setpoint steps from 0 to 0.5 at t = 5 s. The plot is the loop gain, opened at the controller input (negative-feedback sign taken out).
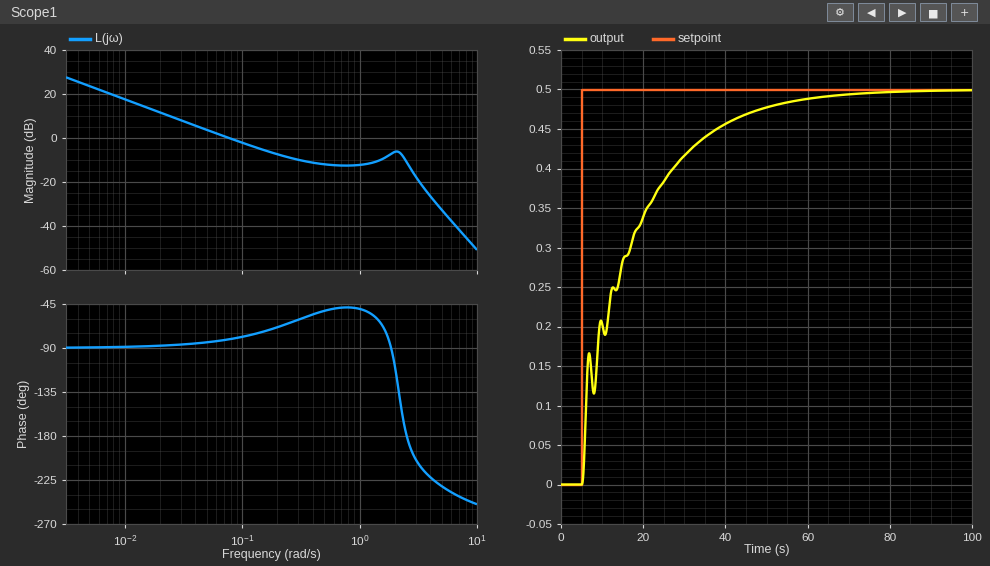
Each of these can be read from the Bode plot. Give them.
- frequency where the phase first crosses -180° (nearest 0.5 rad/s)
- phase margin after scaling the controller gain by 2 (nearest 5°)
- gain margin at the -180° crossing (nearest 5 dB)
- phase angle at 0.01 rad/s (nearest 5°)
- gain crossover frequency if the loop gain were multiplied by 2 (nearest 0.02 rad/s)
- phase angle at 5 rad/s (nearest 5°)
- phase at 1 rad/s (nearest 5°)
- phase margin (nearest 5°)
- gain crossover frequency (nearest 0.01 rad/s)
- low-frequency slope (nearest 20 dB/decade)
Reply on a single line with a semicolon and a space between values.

2.5 rad/s; 110°; 10 dB; -90°; 0.16 rad/s; -230°; -50°; 100°; 0.08 rad/s; -20 dB/decade
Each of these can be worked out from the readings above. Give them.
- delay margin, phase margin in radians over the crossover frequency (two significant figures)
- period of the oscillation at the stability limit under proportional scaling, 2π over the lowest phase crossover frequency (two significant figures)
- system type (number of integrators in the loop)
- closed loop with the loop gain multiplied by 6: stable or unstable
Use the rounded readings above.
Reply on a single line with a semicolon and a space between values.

22 s; 2.5 s; 1; unstable
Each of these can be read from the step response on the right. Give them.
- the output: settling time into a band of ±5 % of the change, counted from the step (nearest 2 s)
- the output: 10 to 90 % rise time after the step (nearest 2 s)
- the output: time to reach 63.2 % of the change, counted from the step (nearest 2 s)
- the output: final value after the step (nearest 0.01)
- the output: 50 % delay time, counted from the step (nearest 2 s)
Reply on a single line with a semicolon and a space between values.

44 s; 32 s; 12 s; 0.50; 8 s
